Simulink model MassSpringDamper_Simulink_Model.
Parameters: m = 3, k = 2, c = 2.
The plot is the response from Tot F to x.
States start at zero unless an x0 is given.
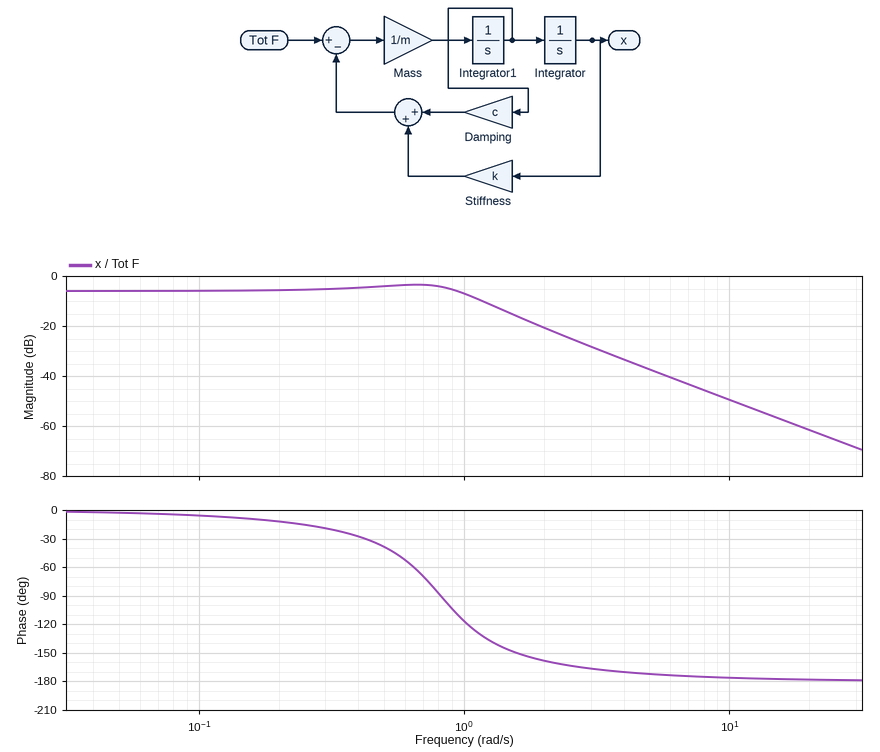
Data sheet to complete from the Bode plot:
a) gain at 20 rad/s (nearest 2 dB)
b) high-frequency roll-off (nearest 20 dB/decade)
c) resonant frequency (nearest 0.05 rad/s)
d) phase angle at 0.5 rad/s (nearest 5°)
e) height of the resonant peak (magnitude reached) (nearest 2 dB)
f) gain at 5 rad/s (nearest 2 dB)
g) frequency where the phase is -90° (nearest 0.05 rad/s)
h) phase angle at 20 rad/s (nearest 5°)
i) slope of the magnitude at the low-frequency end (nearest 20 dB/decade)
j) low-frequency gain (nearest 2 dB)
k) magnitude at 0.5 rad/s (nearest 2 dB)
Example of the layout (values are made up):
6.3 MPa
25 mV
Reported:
-62 dB
-40 dB/decade
0.65 rad/s
-40°
-4 dB
-38 dB
0.80 rad/s
-180°
0 dB/decade
-6 dB
-4 dB
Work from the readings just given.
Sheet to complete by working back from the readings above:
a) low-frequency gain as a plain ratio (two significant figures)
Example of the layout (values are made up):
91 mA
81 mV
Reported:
0.50
